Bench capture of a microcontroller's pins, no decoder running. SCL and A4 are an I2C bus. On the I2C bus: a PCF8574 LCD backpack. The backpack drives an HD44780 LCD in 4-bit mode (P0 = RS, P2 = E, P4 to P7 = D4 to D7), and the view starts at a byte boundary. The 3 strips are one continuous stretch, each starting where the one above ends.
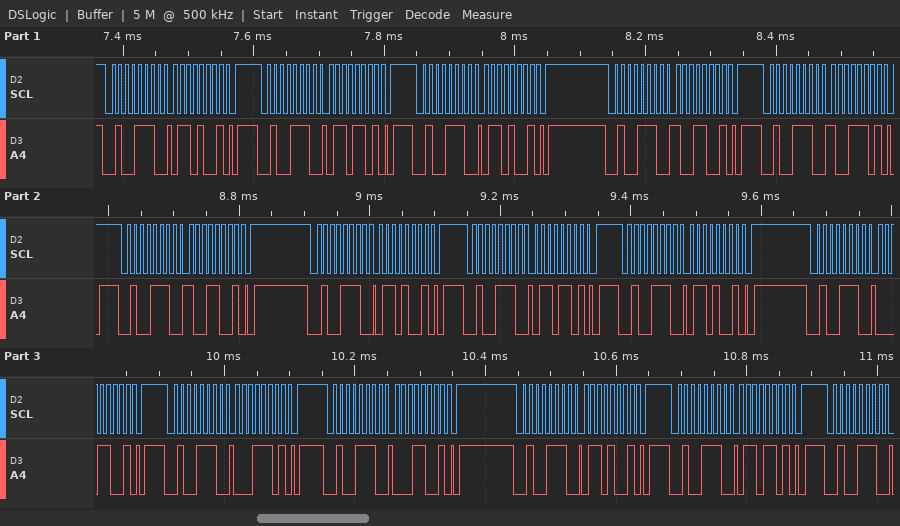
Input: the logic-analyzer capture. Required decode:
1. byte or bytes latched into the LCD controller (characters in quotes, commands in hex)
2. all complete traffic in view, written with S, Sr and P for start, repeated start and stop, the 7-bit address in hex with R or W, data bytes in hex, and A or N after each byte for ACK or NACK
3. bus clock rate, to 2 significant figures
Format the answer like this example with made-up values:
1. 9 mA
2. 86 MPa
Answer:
1. 'i' 'a'
2. S 27W A 69 A P S 27W A 6D A P S 27W A 69 A P S 27W A 99 A P S 27W A 9D A P S 27W A 99 A P S 27W A 69 A P S 27W A 6D A P S 27W A 69 A P S 27W A 19 A P S 27W A 1D A P S 27W A 19 A P S 27W A 69 A P S 27W A 6D A P S 27W A
3. 100 kHz
